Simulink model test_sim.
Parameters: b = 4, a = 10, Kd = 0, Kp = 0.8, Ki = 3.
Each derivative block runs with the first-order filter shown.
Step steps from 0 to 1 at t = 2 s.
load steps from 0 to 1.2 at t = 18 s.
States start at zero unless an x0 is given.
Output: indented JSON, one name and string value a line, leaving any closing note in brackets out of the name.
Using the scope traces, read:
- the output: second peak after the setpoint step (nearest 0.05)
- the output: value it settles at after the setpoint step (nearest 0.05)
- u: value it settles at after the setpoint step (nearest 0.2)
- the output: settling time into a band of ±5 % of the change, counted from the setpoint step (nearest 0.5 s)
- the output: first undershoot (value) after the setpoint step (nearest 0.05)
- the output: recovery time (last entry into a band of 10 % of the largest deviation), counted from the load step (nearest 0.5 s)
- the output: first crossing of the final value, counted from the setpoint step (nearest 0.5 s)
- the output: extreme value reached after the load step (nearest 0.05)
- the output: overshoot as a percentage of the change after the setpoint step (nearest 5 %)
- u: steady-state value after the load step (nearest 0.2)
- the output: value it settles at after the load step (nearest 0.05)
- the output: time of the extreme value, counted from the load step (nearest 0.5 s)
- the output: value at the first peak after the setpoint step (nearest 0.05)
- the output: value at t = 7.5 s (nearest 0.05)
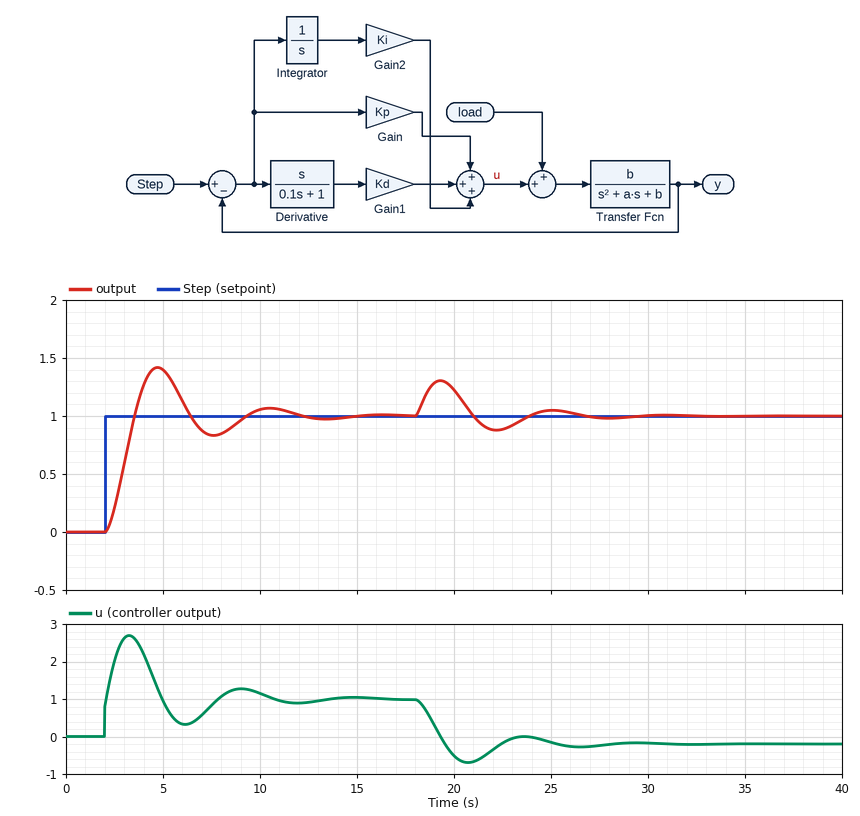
{
  "the output: second peak after the setpoint step": "1.05",
  "the output: value it settles at after the setpoint step": "1.00",
  "u: value it settles at after the setpoint step": "1.0",
  "the output: settling time into a band of ±5 % of the change, counted from the setpoint step": "9.0 s",
  "the output: first undershoot (value) after the setpoint step": "0.85",
  "the output: recovery time (last entry into a band of 10 % of the largest deviation), counted from the load step": "8.0 s",
  "the output: first crossing of the final value, counted from the setpoint step": "1.5 s",
  "the output: extreme value reached after the load step": "1.30",
  "the output: overshoot as a percentage of the change after the setpoint step": "40 %",
  "u: steady-state value after the load step": "-0.2",
  "the output: value it settles at after the load step": "1.00",
  "the output: time of the extreme value, counted from the load step": "1.5 s",
  "the output: value at the first peak after the setpoint step": "1.40",
  "the output: value at t = 7.5 s": "0.85"
}
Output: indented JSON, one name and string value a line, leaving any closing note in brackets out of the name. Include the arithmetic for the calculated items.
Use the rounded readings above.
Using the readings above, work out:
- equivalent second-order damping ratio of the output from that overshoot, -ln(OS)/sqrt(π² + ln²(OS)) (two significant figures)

{
  "equivalent second-order damping ratio of the output from that overshoot, -ln(OS)/sqrt(π² + ln²(OS))": "ln(0.4) = -0.916; 0.916 / sqrt(9.870 + 0.840) = 0.28"
}
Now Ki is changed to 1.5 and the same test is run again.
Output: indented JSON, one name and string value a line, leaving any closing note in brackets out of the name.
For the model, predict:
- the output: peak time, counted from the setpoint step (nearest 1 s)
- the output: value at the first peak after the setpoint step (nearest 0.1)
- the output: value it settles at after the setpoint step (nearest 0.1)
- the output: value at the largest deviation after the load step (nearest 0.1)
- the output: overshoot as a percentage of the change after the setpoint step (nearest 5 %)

{
  "the output: peak time, counted from the setpoint step": "4 s",
  "the output: value at the first peak after the setpoint step": "1.2",
  "the output: value it settles at after the setpoint step": "1.0",
  "the output: value at the largest deviation after the load step": "1.4",
  "the output: overshoot as a percentage of the change after the setpoint step": "25 %"
}
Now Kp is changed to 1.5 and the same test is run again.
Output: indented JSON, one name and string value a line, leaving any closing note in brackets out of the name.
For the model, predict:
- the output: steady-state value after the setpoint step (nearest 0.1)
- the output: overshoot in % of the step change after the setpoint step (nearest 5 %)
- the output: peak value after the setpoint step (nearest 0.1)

{
  "the output: steady-state value after the setpoint step": "1.0",
  "the output: overshoot in % of the step change after the setpoint step": "30 %",
  "the output: peak value after the setpoint step": "1.3"
}
